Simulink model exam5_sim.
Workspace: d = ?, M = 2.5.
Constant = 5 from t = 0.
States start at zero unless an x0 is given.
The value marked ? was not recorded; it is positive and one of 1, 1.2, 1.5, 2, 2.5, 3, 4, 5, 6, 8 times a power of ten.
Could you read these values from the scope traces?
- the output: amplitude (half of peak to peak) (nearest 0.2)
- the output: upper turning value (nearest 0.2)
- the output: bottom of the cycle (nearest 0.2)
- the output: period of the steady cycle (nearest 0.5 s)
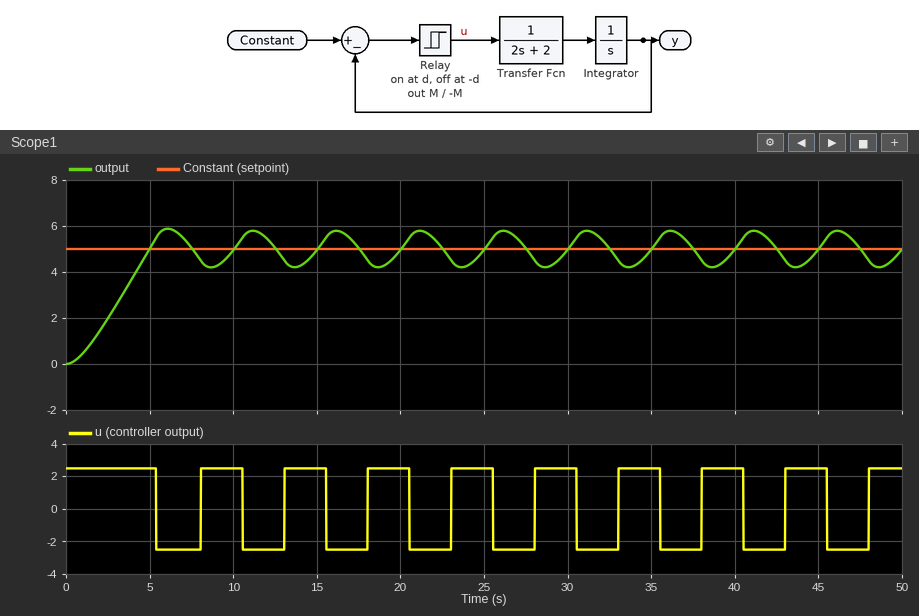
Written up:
0.8
5.8
4.2
5.0 s
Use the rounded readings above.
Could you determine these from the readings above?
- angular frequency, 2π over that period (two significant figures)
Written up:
1.3 rad/s
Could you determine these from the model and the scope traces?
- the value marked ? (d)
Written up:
0.5
